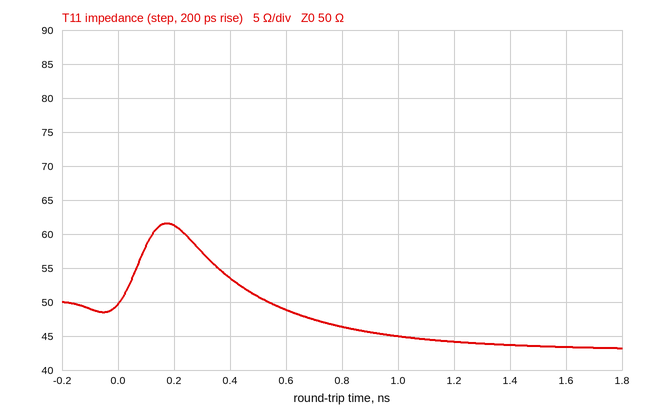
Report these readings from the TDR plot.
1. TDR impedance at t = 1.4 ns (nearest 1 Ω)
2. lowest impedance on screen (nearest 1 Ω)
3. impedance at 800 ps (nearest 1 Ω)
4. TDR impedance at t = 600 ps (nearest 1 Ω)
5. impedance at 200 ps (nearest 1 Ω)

44 Ω
43 Ω
46 Ω
49 Ω
61 Ω
